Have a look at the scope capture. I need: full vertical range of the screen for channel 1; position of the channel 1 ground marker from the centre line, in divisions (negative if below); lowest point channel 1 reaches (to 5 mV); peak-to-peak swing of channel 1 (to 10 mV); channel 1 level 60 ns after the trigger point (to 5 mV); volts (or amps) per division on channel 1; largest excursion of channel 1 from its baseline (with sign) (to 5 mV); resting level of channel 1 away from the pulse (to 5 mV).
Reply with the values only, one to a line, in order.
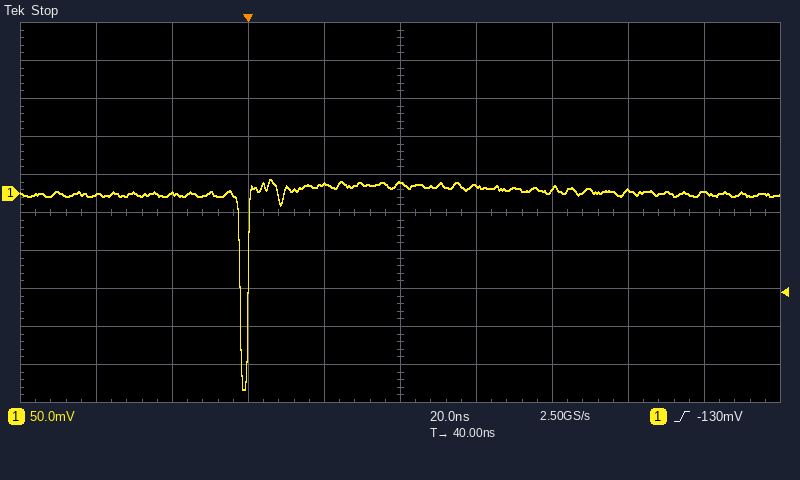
500 mV
+0.5 div
-260 mV
280 mV
10 mV
50 mV
-260 mV
0 mV
